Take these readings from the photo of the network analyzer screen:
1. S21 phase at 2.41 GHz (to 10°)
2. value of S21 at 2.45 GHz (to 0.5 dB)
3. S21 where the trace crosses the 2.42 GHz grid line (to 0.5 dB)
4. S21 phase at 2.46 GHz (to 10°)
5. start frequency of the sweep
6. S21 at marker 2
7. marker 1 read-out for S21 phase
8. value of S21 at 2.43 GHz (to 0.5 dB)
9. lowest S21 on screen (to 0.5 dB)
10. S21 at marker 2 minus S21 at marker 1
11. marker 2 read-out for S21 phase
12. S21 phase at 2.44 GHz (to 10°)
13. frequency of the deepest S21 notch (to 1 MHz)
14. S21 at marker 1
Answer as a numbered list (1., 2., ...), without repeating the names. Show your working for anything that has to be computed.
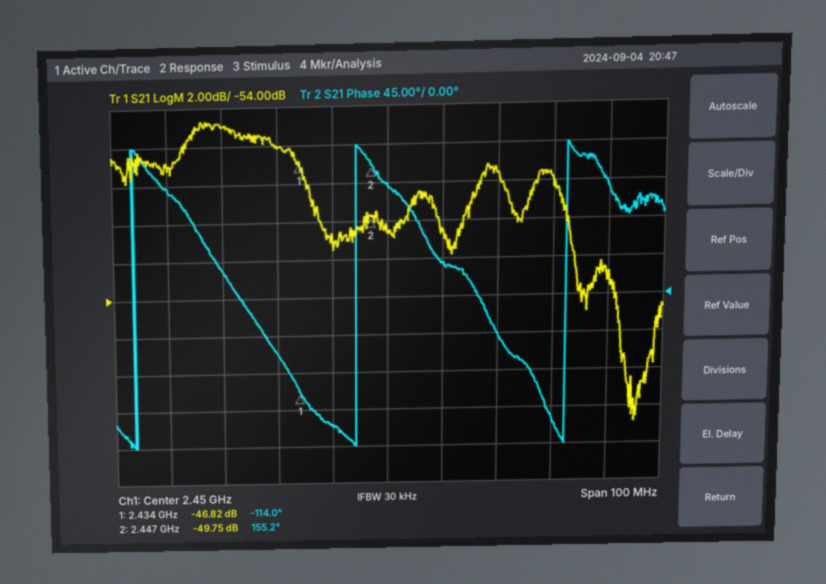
1. 130°
2. -50.5 dB
3. -45.0 dB
4. 40°
5. 2.4 GHz
6. -49.75 dB
7. -114.0°
8. -46.0 dB
9. -61.0 dB
10. -49.75 − (-46.82) = -2.93 dB
11. 155.2°
12. -150°
13. 2.495 GHz
14. -46.82 dB
